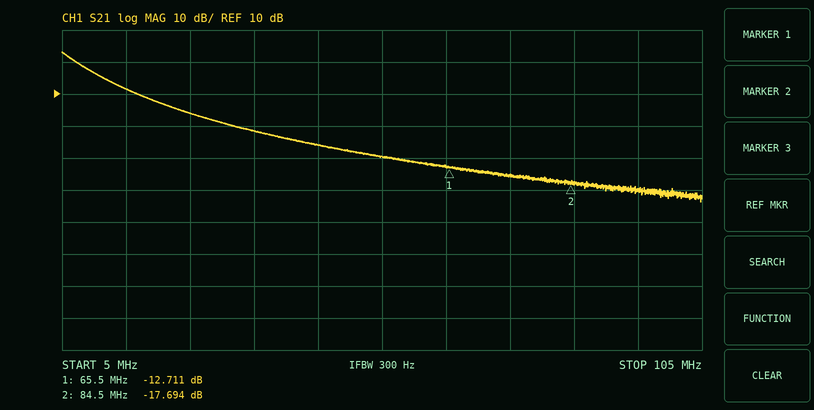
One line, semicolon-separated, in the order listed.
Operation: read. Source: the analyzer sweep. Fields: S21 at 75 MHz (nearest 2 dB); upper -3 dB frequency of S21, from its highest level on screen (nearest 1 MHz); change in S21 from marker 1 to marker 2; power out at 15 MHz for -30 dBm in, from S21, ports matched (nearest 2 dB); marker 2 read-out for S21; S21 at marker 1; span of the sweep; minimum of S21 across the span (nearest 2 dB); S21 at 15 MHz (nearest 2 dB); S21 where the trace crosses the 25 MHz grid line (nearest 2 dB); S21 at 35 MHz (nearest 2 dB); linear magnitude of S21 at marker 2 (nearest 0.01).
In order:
-16 dB; 7 MHz; -4.983 dB; -18 dBm; -17.694 dB; -12.711 dB; 100 MHz; -24 dB; 12 dB; 4 dB; -2 dB; 0.13
